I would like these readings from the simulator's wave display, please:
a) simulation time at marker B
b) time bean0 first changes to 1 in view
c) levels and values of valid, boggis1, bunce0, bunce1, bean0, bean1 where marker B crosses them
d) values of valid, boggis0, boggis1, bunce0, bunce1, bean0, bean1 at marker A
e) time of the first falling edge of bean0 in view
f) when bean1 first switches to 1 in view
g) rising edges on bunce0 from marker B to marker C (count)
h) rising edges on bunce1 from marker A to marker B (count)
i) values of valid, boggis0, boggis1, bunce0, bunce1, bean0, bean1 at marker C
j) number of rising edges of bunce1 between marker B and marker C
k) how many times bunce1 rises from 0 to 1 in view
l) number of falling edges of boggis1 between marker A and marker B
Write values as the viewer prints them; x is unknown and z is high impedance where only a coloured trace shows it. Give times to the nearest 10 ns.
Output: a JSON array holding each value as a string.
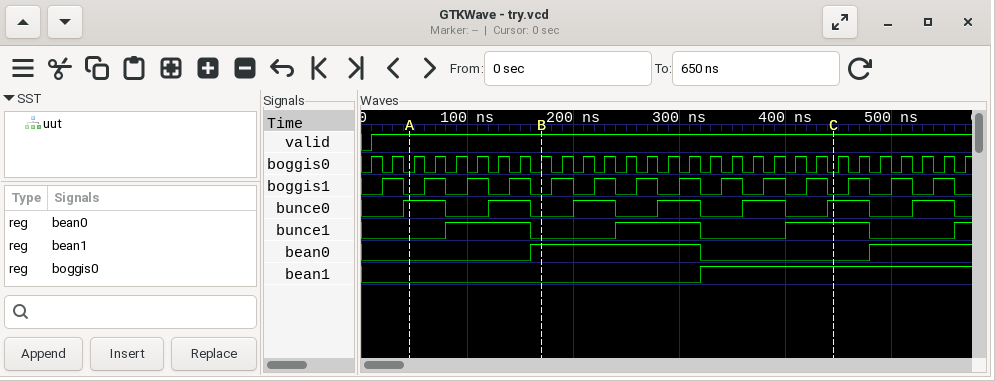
["170 ns", "160 ns", "valid=1, boggis1=0, bunce0=0, bunce1=0, bean0=1, bean1=0", "valid=1, boggis0=0, boggis1=0, bunce0=1, bunce1=0, bean0=0, bean1=0", "320 ns", "320 ns", "4", "1", "valid=1, boggis0=0, boggis1=0, bunce0=1, bunce1=1, bean0=0, bean1=1", "2", "4", "3"]
